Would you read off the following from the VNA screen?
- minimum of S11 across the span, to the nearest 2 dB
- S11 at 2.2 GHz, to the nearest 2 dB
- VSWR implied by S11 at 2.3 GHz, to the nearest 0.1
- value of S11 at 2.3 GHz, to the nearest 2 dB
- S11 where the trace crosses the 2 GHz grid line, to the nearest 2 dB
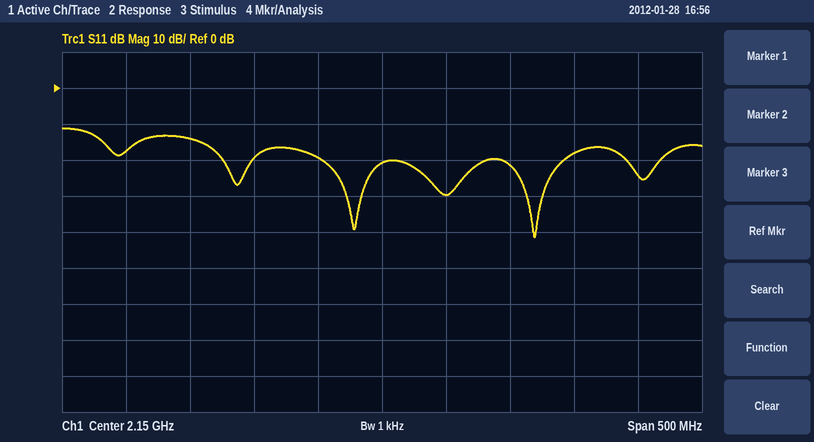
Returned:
-42 dB
-30 dB
1.3
-18 dB
-14 dB
